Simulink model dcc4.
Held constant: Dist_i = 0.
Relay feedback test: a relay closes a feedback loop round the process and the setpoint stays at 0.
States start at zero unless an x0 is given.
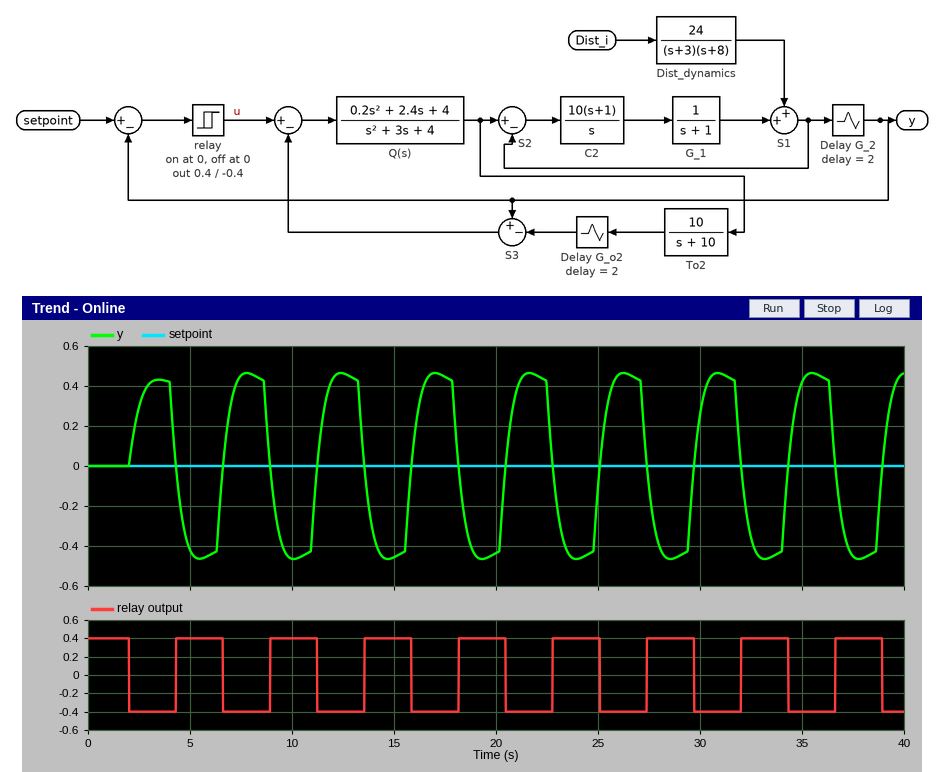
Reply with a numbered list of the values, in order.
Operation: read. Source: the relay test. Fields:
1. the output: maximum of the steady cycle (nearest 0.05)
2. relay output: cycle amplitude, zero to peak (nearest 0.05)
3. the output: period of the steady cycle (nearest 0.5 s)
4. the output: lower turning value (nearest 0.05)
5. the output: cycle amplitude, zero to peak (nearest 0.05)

1. 0.45
2. 0.40
3. 4.5 s
4. -0.45
5. 0.45
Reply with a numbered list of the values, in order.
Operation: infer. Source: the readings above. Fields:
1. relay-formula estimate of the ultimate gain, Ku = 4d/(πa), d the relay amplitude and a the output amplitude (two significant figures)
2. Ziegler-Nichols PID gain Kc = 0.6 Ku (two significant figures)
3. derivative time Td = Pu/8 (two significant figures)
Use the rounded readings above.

1. 1.1
2. 0.66
3. 0.56 s
